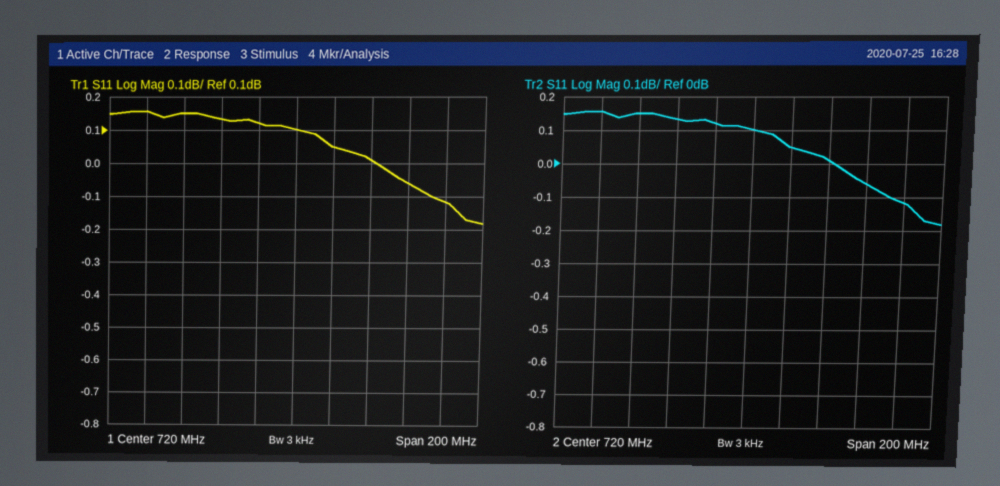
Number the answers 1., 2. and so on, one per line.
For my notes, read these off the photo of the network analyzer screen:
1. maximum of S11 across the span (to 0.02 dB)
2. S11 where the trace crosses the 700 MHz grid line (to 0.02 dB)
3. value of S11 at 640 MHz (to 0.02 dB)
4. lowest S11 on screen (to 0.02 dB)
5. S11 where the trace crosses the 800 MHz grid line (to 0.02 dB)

1. 0.16 dB
2. 0.12 dB
3. 0.16 dB
4. -0.18 dB
5. -0.12 dB
